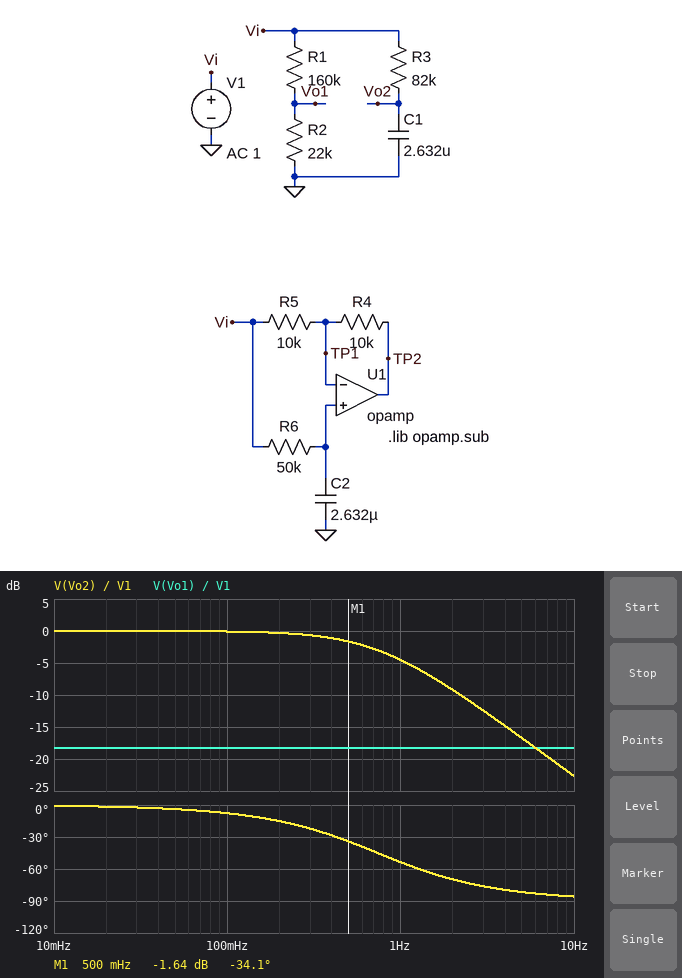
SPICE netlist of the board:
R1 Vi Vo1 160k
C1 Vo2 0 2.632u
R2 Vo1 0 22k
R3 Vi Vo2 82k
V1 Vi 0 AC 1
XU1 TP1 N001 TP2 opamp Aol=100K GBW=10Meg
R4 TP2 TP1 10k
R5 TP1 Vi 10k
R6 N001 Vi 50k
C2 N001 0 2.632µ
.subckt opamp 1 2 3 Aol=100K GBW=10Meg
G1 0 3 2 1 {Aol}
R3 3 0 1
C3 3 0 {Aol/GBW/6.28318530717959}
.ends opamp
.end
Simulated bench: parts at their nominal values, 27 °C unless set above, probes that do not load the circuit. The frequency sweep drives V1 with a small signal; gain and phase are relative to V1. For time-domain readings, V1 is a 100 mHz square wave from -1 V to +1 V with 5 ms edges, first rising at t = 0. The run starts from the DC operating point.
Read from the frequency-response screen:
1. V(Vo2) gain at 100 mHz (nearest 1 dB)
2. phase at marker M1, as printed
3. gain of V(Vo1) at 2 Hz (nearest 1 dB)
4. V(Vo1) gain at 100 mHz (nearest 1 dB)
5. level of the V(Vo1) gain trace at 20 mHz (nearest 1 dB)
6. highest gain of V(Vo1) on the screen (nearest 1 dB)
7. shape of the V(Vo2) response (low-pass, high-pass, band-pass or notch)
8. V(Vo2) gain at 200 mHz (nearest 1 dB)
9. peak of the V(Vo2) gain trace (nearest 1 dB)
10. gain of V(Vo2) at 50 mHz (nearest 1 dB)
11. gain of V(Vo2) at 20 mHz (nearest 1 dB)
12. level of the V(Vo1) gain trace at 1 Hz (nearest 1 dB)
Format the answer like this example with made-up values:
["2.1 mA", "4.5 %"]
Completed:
["0 dB", "-34.1 deg", "-18 dB", "-18 dB", "-18 dB", "-18 dB", "low-pass", "0 dB", "0 dB", "0 dB", "0 dB", "-18 dB"]
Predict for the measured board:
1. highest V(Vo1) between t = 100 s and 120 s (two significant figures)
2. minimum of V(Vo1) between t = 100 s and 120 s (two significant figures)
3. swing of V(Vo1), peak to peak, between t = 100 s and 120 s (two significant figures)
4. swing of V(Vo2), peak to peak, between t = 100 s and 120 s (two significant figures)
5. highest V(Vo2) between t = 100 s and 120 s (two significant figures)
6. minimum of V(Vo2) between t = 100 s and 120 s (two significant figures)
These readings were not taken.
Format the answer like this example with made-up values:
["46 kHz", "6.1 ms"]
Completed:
["120 mV", "-120 mV", "240 mV", "2.0 V", "1.0 V", "-1.0 V"]
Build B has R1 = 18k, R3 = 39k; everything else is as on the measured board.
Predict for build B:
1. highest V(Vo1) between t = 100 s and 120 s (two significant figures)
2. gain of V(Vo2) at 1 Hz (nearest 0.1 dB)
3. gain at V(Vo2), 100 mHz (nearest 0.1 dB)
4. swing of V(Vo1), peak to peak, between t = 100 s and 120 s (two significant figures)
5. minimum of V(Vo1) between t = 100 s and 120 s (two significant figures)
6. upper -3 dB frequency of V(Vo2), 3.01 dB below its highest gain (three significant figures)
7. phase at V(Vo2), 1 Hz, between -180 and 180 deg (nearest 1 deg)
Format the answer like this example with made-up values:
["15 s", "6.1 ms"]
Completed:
["550 mV", "-1.5 dB", "0 dB", "1.1 V", "-550 mV", "1.55 Hz", "-33 deg"]
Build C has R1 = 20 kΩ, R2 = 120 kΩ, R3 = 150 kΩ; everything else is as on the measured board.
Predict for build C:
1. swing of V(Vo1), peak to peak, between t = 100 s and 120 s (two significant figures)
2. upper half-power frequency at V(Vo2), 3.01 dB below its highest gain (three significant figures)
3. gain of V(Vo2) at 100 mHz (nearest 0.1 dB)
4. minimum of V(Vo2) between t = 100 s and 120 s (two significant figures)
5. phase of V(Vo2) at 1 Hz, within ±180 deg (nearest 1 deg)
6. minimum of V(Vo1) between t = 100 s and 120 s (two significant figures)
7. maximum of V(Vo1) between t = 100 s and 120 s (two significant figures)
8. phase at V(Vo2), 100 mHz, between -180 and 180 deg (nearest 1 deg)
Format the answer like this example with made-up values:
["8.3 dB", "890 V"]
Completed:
["1.7 V", "403 mHz", "-0.3 dB", "-1.0 V", "-68 deg", "-860 mV", "860 mV", "-14 deg"]
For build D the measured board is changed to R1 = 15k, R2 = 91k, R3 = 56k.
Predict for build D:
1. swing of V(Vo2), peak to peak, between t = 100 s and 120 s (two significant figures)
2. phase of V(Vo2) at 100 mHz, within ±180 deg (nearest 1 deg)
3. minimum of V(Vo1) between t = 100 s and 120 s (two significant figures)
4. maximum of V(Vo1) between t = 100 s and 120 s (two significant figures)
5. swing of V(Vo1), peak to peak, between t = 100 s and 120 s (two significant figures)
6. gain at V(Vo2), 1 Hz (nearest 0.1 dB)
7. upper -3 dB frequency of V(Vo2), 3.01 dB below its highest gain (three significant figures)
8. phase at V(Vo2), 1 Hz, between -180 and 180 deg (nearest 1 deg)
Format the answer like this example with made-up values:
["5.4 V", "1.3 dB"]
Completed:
["2.0 V", "-5 deg", "-860 mV", "860 mV", "1.7 V", "-2.7 dB", "1.08 Hz", "-43 deg"]
